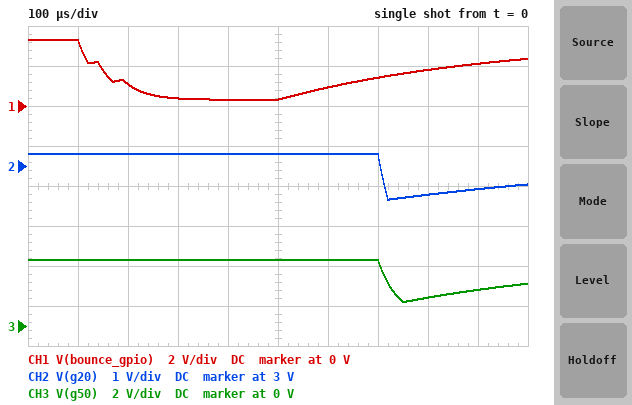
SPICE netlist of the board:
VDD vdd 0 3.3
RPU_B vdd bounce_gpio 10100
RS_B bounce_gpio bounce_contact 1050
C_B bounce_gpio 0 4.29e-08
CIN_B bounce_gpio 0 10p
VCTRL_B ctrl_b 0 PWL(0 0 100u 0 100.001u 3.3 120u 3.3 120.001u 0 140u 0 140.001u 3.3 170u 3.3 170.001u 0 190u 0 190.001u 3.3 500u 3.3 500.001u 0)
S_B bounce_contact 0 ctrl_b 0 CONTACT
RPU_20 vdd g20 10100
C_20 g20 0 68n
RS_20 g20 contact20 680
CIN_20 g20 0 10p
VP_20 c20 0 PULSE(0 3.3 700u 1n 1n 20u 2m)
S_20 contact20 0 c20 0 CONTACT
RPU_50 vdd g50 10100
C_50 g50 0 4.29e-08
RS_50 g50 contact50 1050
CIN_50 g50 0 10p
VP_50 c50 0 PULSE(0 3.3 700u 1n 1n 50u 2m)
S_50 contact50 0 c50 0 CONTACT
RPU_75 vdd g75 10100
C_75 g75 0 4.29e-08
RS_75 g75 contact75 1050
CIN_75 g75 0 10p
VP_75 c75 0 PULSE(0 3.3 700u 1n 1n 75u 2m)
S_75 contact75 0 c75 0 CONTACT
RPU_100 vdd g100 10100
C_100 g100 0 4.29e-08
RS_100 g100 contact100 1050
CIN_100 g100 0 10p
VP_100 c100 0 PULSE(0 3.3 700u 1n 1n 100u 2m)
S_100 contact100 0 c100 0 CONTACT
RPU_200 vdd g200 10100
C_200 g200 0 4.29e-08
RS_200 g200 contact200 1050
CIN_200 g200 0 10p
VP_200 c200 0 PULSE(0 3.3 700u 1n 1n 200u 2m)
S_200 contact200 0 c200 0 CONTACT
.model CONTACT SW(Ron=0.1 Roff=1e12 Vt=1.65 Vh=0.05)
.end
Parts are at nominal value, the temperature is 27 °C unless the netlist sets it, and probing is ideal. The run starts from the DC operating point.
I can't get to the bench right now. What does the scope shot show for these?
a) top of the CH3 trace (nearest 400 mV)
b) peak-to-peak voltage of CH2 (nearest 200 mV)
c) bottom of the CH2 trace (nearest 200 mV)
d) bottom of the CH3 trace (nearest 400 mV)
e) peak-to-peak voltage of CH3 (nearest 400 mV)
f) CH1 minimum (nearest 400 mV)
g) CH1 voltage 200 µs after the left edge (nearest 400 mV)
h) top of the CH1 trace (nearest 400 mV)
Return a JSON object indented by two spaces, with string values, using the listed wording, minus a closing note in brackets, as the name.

{
  "top of the CH3 trace": "3.2 V",
  "peak-to-peak voltage of CH2": "1.2 V",
  "bottom of the CH2 trace": "2.2 V",
  "bottom of the CH3 trace": "1.2 V",
  "peak-to-peak voltage of CH3": "2.0 V",
  "CH1 minimum": "400 mV",
  "CH1 voltage 200 µs after the left edge": "1.2 V",
  "top of the CH1 trace": "3.2 V"
}
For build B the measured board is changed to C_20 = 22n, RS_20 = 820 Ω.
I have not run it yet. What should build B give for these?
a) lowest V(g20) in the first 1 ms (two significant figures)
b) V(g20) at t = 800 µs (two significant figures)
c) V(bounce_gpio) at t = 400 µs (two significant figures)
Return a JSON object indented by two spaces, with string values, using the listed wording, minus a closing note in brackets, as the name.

{
  "lowest V(g20) in the first 1 ms": "1.2 V",
  "V(g20) at t = 800 µs": "1.8 V",
  "V(bounce_gpio) at t = 400 µs": "320 mV"
}
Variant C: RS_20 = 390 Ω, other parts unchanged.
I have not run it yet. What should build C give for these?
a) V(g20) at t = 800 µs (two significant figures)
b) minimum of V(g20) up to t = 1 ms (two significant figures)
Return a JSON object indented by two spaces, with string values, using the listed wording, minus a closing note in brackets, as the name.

{
  "V(g20) at t = 800 µs": "1.8 V",
  "minimum of V(g20) up to t = 1 ms": "1.6 V"
}
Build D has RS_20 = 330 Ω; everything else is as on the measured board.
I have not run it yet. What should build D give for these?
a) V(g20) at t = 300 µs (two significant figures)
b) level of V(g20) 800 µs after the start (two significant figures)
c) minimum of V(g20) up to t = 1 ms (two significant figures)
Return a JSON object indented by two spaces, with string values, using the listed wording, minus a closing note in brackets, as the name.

{
  "V(g20) at t = 300 µs": "3.3 V",
  "level of V(g20) 800 µs after the start": "1.6 V",
  "minimum of V(g20) up to t = 1 ms": "1.4 V"
}
